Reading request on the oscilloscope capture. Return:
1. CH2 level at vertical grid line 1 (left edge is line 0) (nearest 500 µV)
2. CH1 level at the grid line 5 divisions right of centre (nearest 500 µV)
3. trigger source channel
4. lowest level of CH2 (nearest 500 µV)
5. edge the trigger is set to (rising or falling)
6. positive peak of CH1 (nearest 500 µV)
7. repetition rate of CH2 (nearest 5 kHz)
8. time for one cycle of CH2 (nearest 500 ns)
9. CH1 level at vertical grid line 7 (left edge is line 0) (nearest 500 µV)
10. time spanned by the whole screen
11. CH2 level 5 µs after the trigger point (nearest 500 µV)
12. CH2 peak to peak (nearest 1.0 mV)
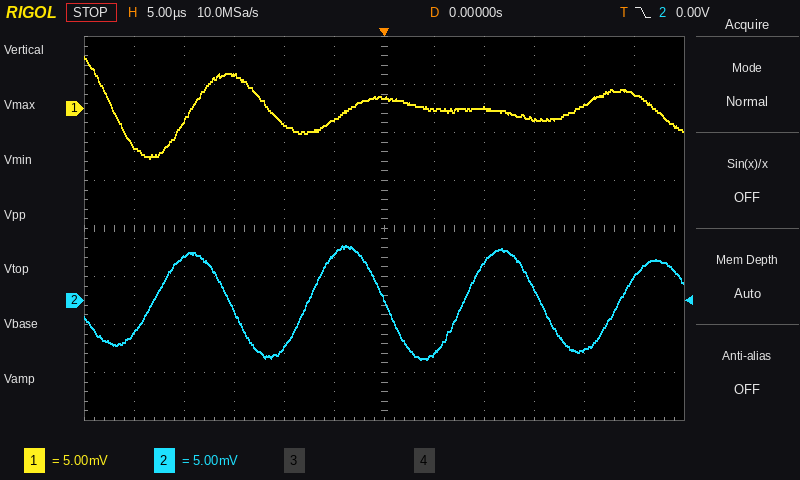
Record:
-3.5 mV
1.5 mV
CH2
-6.0 mV
falling
5.5 mV
65 kHz
15.5 µs
0.0 mV
60 µs
-5.5 mV
12.0 mV
